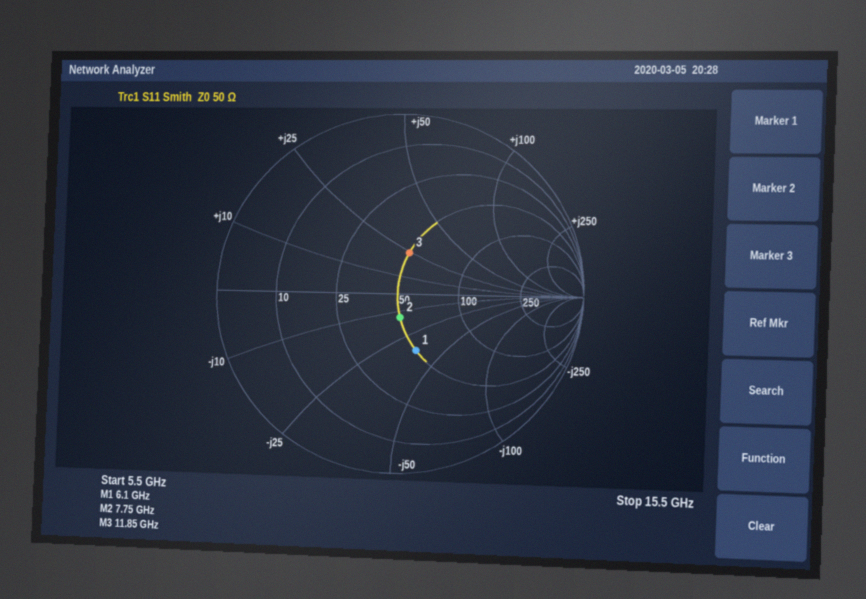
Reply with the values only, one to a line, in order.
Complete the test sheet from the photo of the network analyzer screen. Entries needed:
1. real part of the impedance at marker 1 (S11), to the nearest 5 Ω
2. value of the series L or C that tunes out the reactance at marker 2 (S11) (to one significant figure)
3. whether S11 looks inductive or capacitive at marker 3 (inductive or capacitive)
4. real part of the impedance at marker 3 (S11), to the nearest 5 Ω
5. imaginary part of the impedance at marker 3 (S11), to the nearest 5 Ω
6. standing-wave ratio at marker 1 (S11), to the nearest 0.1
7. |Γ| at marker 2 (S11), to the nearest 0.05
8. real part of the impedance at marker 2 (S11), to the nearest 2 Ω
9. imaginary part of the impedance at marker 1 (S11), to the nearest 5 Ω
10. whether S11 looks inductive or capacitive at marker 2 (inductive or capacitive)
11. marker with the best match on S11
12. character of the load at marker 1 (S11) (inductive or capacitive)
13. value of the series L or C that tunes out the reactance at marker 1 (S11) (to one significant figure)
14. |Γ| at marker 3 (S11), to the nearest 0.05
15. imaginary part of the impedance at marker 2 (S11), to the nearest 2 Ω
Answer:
50 Ω
300 pH
inductive
50 Ω
+25 Ω
2.0
0.15
50 Ω
-35 Ω
capacitive
marker 2
capacitive
900 pH
0.25
-14 Ω
